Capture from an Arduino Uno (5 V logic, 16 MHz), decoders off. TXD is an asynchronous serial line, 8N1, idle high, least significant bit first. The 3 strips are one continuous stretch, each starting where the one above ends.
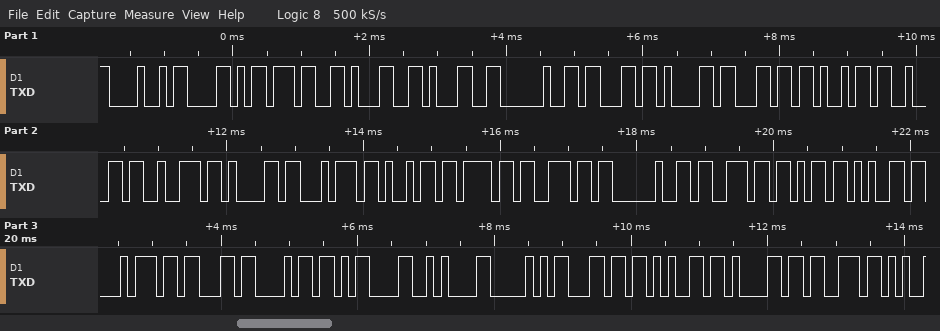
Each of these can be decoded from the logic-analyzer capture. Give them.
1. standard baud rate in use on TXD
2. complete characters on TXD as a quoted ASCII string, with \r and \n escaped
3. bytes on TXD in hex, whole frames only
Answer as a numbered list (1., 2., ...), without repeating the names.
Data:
1. 9600 baud
2. "HX711 calibration sketch\r\nPleas"
3. 48 58 37 31 31 20 63 61 6C 69 62 72 61 74 69 6F 6E 20 73 6B 65 74 63 68 0D 0A 50 6C 65 61 73
